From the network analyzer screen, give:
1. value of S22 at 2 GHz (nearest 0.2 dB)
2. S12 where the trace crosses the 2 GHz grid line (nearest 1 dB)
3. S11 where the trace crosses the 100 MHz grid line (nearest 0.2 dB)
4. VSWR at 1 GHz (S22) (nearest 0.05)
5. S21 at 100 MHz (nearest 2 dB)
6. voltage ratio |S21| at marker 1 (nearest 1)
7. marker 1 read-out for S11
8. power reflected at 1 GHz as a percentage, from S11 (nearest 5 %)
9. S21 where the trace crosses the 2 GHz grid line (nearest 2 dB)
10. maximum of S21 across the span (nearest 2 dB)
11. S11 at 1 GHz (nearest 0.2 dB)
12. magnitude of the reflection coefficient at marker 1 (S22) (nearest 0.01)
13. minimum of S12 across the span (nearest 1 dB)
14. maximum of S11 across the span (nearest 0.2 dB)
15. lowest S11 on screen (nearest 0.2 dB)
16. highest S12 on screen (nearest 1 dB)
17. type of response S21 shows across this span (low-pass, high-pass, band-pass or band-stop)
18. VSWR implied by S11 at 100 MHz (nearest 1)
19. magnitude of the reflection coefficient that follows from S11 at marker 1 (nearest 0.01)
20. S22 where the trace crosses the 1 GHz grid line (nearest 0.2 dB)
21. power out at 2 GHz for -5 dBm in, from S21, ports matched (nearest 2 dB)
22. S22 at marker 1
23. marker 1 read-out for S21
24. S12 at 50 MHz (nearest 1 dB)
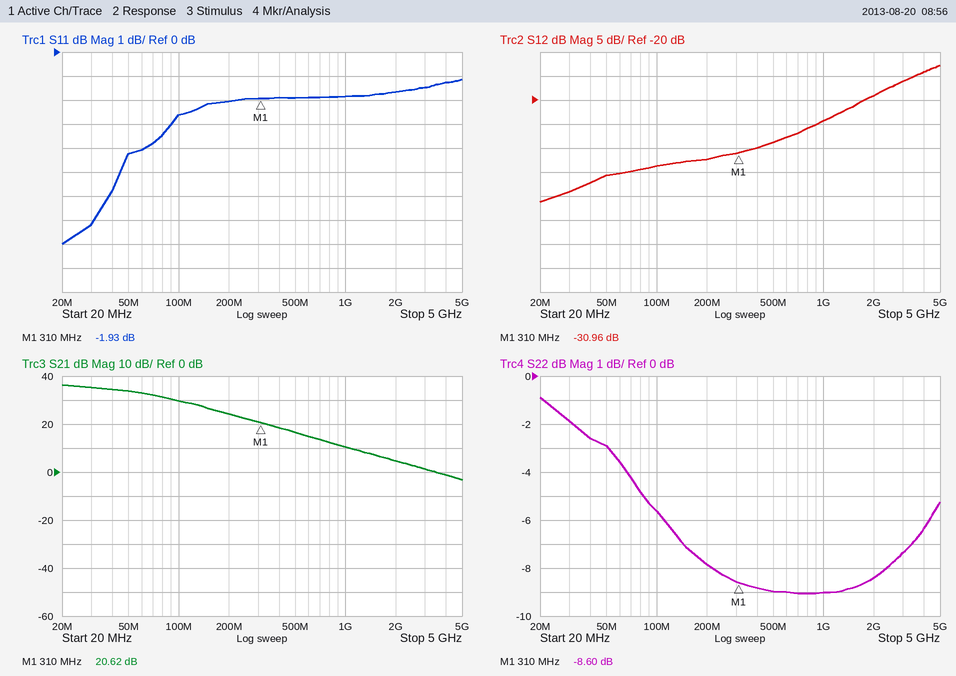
-8.4 dB
-19 dB
-2.6 dB
2.10
30 dB
11
-1.93 dB
65 %
4 dB
36 dB
-1.8 dB
0.37
-41 dB
-1.2 dB
-8.0 dB
-13 dB
low-pass
7
0.80
-9.0 dB
0 dBm
-8.60 dB
20.62 dB
-36 dB
